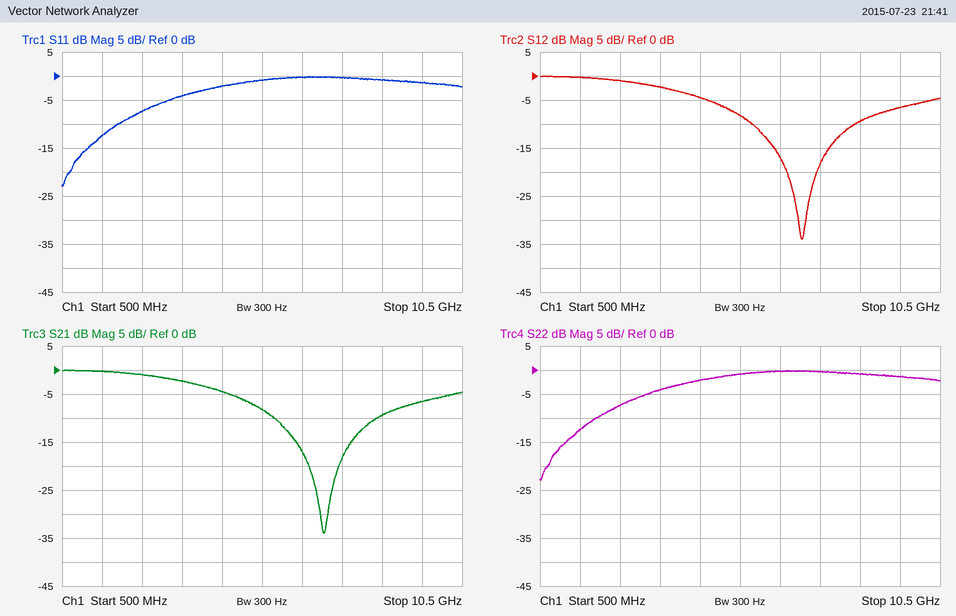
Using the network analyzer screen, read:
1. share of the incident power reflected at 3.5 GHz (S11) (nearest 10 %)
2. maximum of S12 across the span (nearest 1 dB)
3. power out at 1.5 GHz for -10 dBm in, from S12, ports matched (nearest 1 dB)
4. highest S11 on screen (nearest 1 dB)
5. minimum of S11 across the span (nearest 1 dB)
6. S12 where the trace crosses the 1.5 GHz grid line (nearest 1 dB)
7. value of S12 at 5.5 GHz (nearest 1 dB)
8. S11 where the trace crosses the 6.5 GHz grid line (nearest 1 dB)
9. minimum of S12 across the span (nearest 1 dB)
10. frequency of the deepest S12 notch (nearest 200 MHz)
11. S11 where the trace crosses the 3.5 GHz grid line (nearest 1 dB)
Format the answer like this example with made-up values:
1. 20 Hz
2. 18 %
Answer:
1. 40 %
2. 0 dB
3. -10 dBm
4. 0 dB
5. -23 dB
6. 0 dB
7. -8 dB
8. 0 dB
9. -34 dB
10. 7.0 GHz
11. -4 dB
